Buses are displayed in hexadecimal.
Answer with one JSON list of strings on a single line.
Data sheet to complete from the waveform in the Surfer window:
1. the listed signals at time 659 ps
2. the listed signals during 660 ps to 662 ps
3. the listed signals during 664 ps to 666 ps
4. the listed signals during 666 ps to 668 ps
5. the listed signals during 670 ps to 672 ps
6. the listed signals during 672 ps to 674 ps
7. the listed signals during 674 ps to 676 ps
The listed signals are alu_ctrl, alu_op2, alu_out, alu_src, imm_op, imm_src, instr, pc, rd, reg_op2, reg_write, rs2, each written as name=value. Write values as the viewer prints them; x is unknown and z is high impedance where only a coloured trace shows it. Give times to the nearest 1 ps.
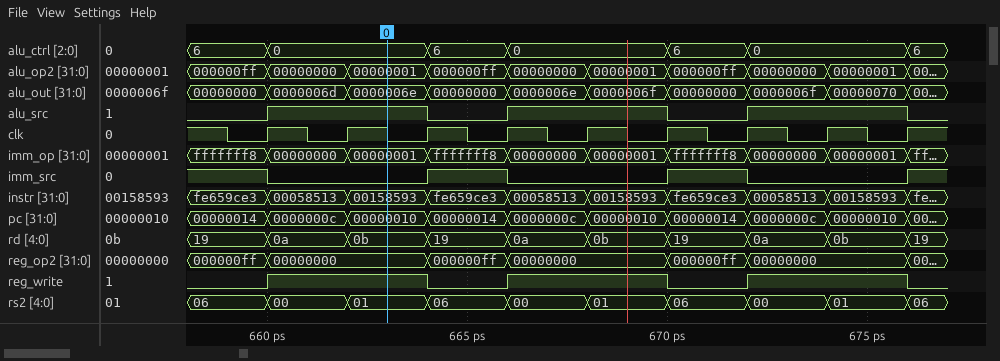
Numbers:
["alu_ctrl=6, alu_op2=000000ff, alu_out=00000000, alu_src=0, imm_op=fffffff8, imm_src=1, instr=fe659ce3, pc=00000014, rd=19, reg_op2=000000ff, reg_write=0, rs2=06", "alu_ctrl=0, alu_op2=00000000, alu_out=0000006d, alu_src=1, imm_op=00000000, imm_src=0, instr=00058513, pc=0000000c, rd=0a, reg_op2=00000000, reg_write=1, rs2=00", "alu_ctrl=6, alu_op2=000000ff, alu_out=00000000, alu_src=0, imm_op=fffffff8, imm_src=1, instr=fe659ce3, pc=00000014, rd=19, reg_op2=000000ff, reg_write=0, rs2=06", "alu_ctrl=0, alu_op2=00000000, alu_out=0000006e, alu_src=1, imm_op=00000000, imm_src=0, instr=00058513, pc=0000000c, rd=0a, reg_op2=00000000, reg_write=1, rs2=00", "alu_ctrl=6, alu_op2=000000ff, alu_out=00000000, alu_src=0, imm_op=fffffff8, imm_src=1, instr=fe659ce3, pc=00000014, rd=19, reg_op2=000000ff, reg_write=0, rs2=06", "alu_ctrl=0, alu_op2=00000000, alu_out=0000006f, alu_src=1, imm_op=00000000, imm_src=0, instr=00058513, pc=0000000c, rd=0a, reg_op2=00000000, reg_write=1, rs2=00", "alu_ctrl=0, alu_op2=00000001, alu_out=00000070, alu_src=1, imm_op=00000001, imm_src=0, instr=00158593, pc=00000010, rd=0b, reg_op2=00000000, reg_write=1, rs2=01"]
